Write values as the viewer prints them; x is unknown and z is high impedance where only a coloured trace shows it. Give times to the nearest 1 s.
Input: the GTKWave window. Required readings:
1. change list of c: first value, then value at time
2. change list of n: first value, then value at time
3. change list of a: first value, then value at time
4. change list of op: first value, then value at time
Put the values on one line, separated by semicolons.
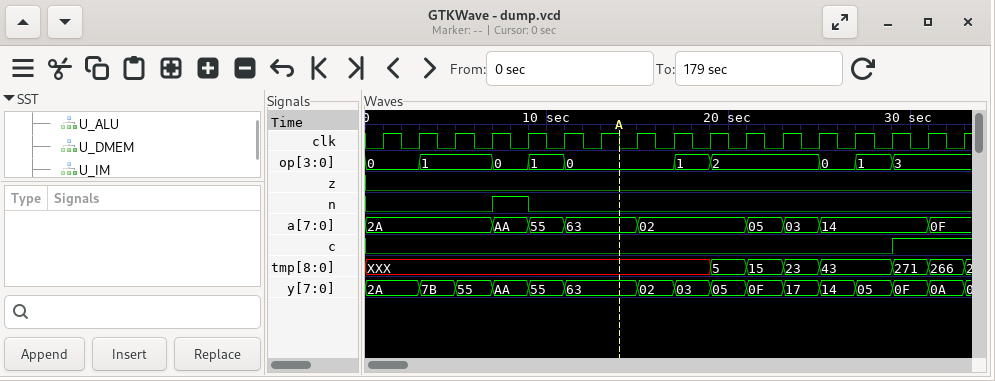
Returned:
0, 1 at 29 s; 0, 1 at 7 s, 0 at 9 s; 2A, AA at 7 s, 55 at 9 s, 63 at 11 s, 02 at 15 s, 05 at 21 s, 03 at 23 s, 14 at 25 s, 0F at 31 s; 0, 1 at 3 s, 0 at 7 s, 1 at 9 s, 0 at 11 s, 1 at 17 s, 2 at 19 s, 0 at 25 s, 1 at 27 s, 3 at 29 s
